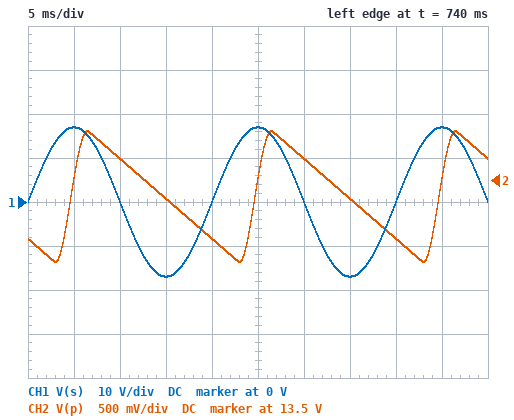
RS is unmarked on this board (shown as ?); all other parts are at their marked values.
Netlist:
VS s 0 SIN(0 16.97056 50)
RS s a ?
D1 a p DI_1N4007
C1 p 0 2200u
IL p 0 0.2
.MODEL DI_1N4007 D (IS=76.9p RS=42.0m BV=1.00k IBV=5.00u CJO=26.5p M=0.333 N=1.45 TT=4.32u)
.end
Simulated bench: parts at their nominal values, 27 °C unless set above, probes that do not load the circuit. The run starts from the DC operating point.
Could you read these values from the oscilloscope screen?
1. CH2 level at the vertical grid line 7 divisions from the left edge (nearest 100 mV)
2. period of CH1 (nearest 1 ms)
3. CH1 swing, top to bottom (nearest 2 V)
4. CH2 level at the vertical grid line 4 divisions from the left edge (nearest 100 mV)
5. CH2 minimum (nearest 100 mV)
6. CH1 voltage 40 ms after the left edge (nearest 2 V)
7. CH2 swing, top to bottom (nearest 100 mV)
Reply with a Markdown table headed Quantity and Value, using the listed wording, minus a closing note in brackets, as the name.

| Quantity | Value |
|---|---|
| CH2 level at the vertical grid line 7 divisions from the left edge | 13.3 V |
| period of CH1 | 20 ms |
| CH1 swing, top to bottom | 34 V |
| CH2 level at the vertical grid line 4 divisions from the left edge | 12.8 V |
| CH2 minimum | 12.6 V |
| CH1 voltage 40 ms after the left edge | 0 V |
| CH2 swing, top to bottom | 1.5 V |
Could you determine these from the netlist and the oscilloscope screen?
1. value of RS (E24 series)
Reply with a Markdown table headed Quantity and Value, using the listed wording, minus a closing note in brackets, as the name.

| Quantity | Value |
|---|---|
| value of RS | 1.6 Ω |
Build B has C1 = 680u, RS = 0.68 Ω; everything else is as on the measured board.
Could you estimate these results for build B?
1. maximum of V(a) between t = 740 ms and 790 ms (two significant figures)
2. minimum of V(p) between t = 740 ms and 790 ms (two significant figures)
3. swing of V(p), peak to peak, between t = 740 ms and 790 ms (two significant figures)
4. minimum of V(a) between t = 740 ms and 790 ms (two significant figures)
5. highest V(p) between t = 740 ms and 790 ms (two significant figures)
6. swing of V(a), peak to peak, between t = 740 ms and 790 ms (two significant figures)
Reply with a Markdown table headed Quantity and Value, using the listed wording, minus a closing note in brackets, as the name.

| Quantity | Value |
|---|---|
| maximum of V(a) between t = 740 ms and 790 ms | 17 V |
| minimum of V(p) between t = 740 ms and 790 ms | 11 V |
| swing of V(p), peak to peak, between t = 740 ms and 790 ms | 4.9 V |
| minimum of V(a) between t = 740 ms and 790 ms | -17 V |
| highest V(p) between t = 740 ms and 790 ms | 16 V |
| swing of V(a), peak to peak, between t = 740 ms and 790 ms | 34 V |
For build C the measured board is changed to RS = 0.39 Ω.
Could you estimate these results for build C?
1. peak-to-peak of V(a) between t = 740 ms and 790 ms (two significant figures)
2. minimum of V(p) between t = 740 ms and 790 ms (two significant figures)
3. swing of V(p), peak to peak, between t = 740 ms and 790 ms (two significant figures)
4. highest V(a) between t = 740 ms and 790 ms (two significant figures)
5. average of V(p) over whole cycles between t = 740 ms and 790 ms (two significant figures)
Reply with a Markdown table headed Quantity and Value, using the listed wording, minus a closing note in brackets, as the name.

| Quantity | Value |
|---|---|
| peak-to-peak of V(a) between t = 740 ms and 790 ms | 33 V |
| minimum of V(p) between t = 740 ms and 790 ms | 14 V |
| swing of V(p), peak to peak, between t = 740 ms and 790 ms | 1.6 V |
| highest V(a) between t = 740 ms and 790 ms | 16 V |
| average of V(p) over whole cycles between t = 740 ms and 790 ms | 15 V |
